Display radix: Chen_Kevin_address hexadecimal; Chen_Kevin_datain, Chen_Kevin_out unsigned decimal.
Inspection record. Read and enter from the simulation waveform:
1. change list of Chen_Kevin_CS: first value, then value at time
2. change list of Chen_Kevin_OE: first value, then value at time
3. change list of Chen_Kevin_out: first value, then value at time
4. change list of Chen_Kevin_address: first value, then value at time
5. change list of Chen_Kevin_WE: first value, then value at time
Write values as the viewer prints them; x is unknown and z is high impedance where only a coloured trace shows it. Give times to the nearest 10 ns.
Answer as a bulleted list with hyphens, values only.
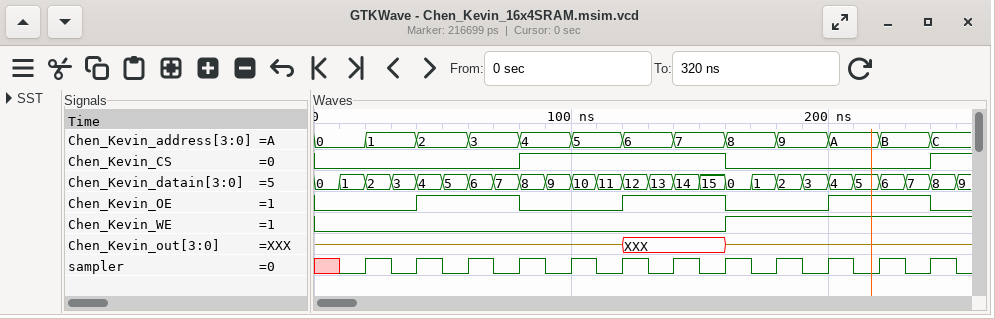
- 0, 1 at 80 ns, 0 at 160 ns, 1 at 240 ns
- 0, 1 at 40 ns, 0 at 80 ns, 1 at 120 ns, 0 at 160 ns, 1 at 200 ns, 0 at 240 ns
- z, XXX at 120 ns, z at 160 ns
- 0, 1 at 20 ns, 2 at 40 ns, 3 at 60 ns, 4 at 80 ns, 5 at 100 ns, 6 at 120 ns, 7 at 140 ns, 8 at 160 ns, 9 at 180 ns, A at 200 ns, B at 220 ns, C at 240 ns
- 0, 1 at 160 ns
